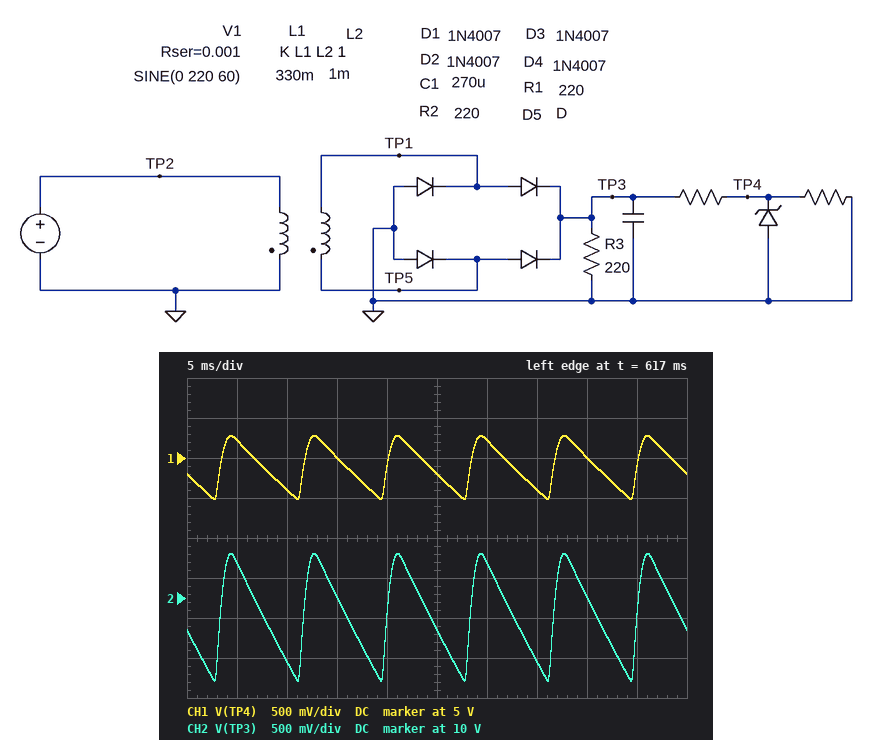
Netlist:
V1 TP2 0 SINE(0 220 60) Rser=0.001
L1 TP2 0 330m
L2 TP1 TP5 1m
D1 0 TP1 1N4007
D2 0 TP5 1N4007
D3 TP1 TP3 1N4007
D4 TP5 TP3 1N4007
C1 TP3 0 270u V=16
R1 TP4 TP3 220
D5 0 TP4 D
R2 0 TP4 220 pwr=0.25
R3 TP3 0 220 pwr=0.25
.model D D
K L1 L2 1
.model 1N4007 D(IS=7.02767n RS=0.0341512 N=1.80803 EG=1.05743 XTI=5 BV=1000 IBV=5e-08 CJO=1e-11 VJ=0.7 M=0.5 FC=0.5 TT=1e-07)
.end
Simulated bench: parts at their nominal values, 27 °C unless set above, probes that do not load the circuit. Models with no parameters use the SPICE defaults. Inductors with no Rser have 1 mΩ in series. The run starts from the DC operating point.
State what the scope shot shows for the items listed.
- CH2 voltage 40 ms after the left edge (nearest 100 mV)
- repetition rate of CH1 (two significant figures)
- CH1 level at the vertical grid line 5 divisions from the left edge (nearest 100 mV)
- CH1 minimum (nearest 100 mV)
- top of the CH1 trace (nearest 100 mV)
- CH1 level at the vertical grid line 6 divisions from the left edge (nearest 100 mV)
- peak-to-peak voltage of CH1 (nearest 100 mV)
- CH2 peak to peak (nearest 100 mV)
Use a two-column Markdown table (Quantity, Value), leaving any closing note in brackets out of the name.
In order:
| Quantity | Value |
|---|---|
| CH2 voltage 40 ms after the left edge | 10.0 V |
| repetition rate of CH1 | 120 Hz |
| CH1 level at the vertical grid line 5 divisions from the left edge | 4.8 V |
| CH1 minimum | 4.5 V |
| top of the CH1 trace | 5.3 V |
| CH1 level at the vertical grid line 6 divisions from the left edge | 5.2 V |
| peak-to-peak voltage of CH1 | 800 mV |
| CH2 peak to peak | 1.6 V |
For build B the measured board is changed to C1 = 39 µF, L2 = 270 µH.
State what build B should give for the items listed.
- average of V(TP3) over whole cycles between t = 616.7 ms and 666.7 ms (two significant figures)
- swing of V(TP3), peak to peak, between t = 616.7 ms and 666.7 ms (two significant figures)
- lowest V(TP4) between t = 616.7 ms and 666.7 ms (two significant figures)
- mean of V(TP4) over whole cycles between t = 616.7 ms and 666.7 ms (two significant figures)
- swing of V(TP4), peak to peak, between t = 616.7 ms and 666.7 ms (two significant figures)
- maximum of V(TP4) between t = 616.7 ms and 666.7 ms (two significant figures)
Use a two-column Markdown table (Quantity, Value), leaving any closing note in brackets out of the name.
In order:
| Quantity | Value |
|---|---|
| average of V(TP3) over whole cycles between t = 616.7 ms and 666.7 ms | 3.5 V |
| swing of V(TP3), peak to peak, between t = 616.7 ms and 666.7 ms | 2.8 V |
| lowest V(TP4) between t = 616.7 ms and 666.7 ms | 1.0 V |
| mean of V(TP4) over whole cycles between t = 616.7 ms and 666.7 ms | 1.8 V |
| swing of V(TP4), peak to peak, between t = 616.7 ms and 666.7 ms | 1.4 V |
| maximum of V(TP4) between t = 616.7 ms and 666.7 ms | 2.4 V |
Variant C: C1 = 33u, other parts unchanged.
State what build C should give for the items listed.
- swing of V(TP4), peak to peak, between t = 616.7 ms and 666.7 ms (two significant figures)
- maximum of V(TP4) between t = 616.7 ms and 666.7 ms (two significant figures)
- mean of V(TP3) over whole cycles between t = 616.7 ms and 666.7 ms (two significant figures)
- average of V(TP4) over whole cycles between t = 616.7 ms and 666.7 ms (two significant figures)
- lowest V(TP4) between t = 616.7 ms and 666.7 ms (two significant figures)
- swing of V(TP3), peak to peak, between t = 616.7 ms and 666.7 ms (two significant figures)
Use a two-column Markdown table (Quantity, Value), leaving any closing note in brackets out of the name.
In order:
| Quantity | Value |
|---|---|
| swing of V(TP4), peak to peak, between t = 616.7 ms and 666.7 ms | 3.3 V |
| maximum of V(TP4) between t = 616.7 ms and 666.7 ms | 5.3 V |
| mean of V(TP3) over whole cycles between t = 616.7 ms and 666.7 ms | 7.6 V |
| average of V(TP4) over whole cycles between t = 616.7 ms and 666.7 ms | 3.8 V |
| lowest V(TP4) between t = 616.7 ms and 666.7 ms | 2.0 V |
| swing of V(TP3), peak to peak, between t = 616.7 ms and 666.7 ms | 6.5 V |
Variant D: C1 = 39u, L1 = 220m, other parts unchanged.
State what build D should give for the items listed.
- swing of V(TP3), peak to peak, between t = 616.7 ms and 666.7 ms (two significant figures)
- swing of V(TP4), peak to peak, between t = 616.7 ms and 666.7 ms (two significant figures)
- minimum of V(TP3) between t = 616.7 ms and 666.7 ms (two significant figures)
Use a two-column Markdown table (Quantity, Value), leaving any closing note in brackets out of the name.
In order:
| Quantity | Value |
|---|---|
| swing of V(TP3), peak to peak, between t = 616.7 ms and 666.7 ms | 7.6 V |
| swing of V(TP4), peak to peak, between t = 616.7 ms and 666.7 ms | 3.8 V |
| minimum of V(TP3) between t = 616.7 ms and 666.7 ms | 5.7 V |
